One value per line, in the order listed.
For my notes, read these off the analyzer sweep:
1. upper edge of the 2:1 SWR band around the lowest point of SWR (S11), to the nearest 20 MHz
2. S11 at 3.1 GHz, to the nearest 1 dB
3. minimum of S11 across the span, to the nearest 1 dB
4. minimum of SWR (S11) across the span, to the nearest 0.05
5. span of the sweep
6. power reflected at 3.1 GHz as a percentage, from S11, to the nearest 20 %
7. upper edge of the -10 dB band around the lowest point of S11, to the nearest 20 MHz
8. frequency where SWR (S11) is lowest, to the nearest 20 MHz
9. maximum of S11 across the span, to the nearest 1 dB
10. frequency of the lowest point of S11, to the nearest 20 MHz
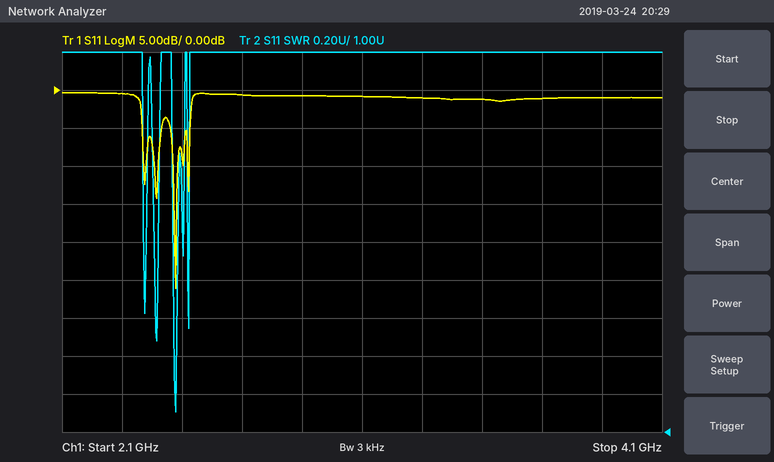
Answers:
2.48 GHz
-1 dB
-26 dB
1.10
2 GHz
80 %
2.48 GHz
2.48 GHz
0 dB
2.48 GHz
